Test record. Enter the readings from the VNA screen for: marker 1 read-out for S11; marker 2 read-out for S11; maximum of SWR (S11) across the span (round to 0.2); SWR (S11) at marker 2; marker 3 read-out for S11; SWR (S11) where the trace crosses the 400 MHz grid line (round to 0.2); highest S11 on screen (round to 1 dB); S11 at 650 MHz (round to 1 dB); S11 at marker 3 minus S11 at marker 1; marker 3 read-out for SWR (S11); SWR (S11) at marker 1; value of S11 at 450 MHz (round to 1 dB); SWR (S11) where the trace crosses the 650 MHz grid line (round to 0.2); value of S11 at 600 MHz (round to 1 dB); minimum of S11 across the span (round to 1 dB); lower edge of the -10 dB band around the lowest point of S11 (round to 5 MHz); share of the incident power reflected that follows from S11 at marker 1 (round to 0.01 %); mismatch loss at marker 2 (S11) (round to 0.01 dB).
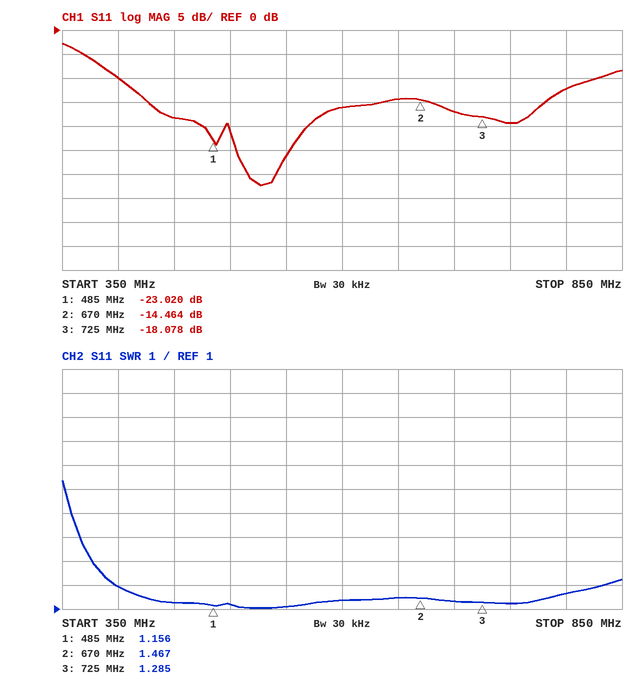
-23.020 dB
-14.464 dB
6.4
1.467
-18.078 dB
2.0
-3 dB
-14 dB
4.942 dB
1.285
1.156
-18 dB
1.4
-16 dB
-32 dB
400 MHz
0.50 %
0.16 dB
